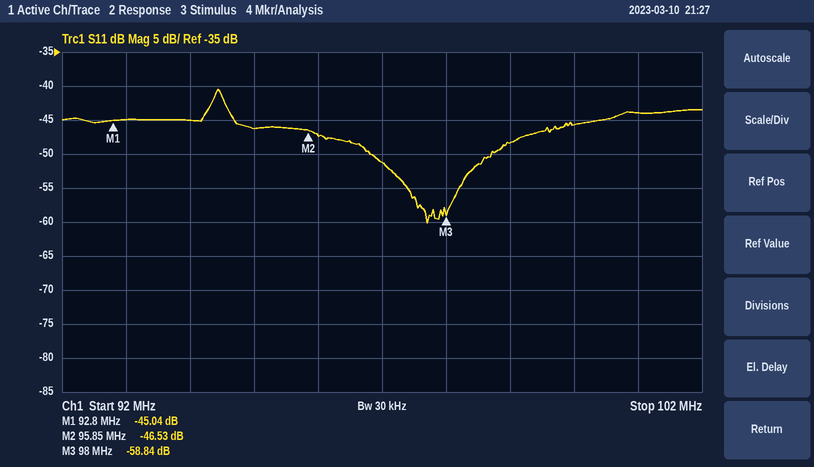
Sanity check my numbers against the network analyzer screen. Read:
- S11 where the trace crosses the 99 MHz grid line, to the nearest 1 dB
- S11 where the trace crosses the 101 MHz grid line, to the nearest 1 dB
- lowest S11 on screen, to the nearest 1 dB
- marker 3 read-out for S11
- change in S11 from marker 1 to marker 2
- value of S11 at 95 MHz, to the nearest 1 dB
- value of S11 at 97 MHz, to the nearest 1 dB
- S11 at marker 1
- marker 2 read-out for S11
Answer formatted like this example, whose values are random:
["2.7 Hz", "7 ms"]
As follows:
["-48 dB", "-44 dB", "-60 dB", "-58.84 dB", "-1.49 dB", "-46 dB", "-51 dB", "-45.04 dB", "-46.53 dB"]
